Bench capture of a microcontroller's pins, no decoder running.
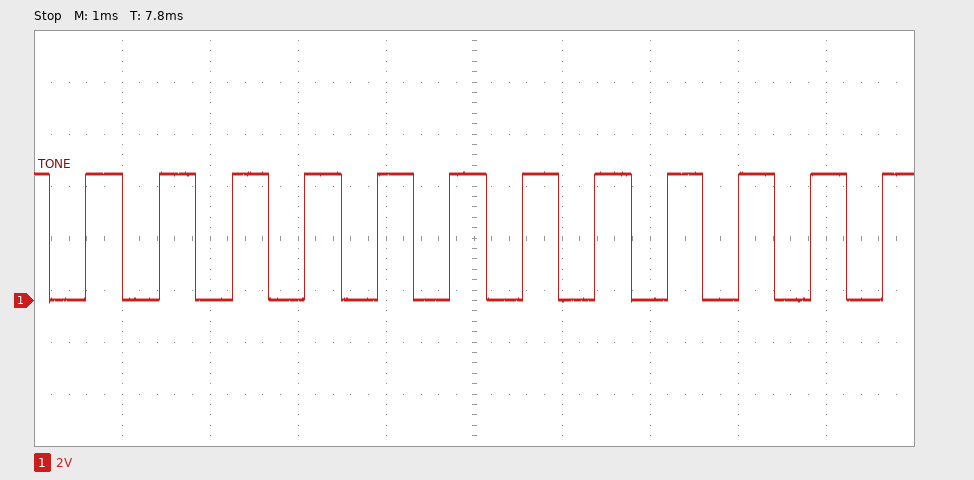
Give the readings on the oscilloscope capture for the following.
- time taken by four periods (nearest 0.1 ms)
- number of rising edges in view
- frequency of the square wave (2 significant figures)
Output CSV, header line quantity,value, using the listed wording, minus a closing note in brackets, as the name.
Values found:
quantity,value
time taken by four periods,3.3 ms
number of rising edges in view,12
frequency of the square wave,1.2 kHz
